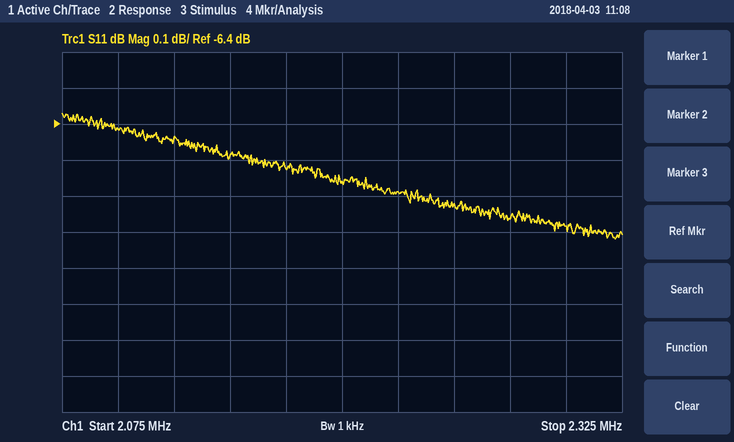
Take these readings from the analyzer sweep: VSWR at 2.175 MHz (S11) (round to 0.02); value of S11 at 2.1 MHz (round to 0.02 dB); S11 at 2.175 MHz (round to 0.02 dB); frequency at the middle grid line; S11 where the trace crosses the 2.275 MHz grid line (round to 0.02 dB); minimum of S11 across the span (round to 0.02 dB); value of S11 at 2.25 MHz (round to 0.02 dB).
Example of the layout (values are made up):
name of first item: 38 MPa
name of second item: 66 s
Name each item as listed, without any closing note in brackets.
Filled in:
VSWR at 2.175 MHz (S11): 2.78
value of S11 at 2.1 MHz: -6.42 dB
S11 at 2.175 MHz: -6.52 dB
frequency at the middle grid line: 2.2 MHz
S11 where the trace crosses the 2.275 MHz grid line: -6.66 dB
minimum of S11 across the span: -6.72 dB
value of S11 at 2.25 MHz: -6.62 dB
